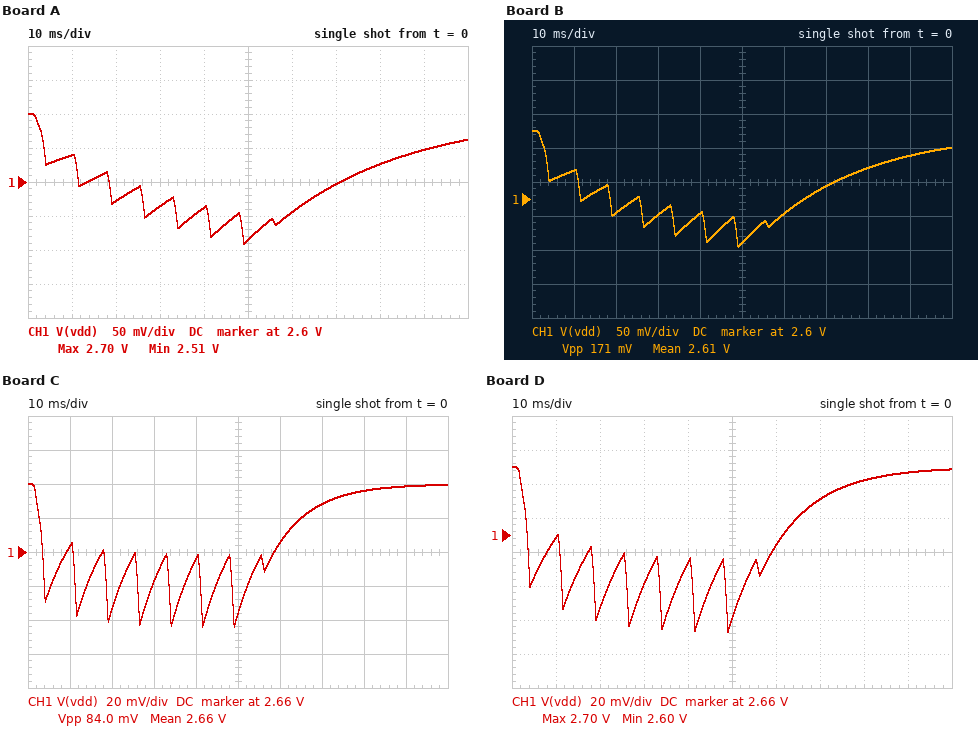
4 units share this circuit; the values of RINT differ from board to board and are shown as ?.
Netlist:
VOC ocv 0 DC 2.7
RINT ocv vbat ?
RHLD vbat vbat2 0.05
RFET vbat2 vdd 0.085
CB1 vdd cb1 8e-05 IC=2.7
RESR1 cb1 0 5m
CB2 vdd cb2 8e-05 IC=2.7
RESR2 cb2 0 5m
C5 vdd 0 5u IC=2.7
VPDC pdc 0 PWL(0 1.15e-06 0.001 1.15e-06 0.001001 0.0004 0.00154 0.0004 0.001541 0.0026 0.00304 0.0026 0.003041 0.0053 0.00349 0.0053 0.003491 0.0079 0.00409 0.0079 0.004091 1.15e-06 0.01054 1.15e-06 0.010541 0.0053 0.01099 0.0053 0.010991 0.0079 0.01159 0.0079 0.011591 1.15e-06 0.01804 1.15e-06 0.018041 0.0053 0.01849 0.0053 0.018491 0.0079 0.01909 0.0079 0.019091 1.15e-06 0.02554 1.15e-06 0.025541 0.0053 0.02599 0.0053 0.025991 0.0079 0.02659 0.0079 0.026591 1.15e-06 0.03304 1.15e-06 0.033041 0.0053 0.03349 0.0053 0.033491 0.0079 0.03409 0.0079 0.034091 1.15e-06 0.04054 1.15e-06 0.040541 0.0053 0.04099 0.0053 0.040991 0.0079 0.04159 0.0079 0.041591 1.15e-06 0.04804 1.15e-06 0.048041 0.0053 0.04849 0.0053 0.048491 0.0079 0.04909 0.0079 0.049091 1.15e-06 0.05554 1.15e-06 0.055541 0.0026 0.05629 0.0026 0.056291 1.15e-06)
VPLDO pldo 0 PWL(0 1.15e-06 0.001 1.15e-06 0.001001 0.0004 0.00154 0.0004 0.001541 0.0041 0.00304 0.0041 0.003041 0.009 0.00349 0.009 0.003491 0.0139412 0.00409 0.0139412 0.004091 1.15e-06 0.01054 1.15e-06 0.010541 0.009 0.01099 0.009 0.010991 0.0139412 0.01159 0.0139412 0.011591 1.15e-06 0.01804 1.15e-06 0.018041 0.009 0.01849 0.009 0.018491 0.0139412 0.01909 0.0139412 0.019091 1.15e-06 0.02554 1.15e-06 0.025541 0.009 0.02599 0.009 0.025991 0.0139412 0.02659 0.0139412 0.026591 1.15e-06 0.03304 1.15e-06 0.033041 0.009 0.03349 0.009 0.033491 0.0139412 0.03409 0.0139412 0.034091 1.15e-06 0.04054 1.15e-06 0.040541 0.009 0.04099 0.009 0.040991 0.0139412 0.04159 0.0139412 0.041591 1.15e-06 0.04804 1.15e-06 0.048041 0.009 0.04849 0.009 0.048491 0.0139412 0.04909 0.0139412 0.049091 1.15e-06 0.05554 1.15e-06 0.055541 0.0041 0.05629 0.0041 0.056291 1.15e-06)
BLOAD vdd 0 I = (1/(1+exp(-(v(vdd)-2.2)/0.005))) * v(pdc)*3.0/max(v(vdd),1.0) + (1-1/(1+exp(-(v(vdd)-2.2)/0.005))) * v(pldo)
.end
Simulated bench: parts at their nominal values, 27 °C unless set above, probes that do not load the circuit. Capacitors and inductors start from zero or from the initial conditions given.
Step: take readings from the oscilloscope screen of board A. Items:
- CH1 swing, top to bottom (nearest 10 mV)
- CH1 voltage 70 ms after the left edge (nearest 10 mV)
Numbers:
190 mV
2.60 V
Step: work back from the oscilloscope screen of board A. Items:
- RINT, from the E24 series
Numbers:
180 Ω
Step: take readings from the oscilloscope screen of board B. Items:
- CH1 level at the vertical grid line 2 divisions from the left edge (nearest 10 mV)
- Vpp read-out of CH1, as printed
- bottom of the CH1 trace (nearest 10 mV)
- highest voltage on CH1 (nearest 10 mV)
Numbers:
2.58 V
171 mV
2.53 V
2.70 V
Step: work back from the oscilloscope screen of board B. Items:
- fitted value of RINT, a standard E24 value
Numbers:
150 Ω
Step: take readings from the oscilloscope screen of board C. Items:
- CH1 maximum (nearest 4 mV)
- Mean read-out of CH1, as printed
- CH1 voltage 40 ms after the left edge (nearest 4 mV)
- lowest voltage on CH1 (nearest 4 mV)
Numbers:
2.700 V
2.66 V
2.656 V
2.616 V
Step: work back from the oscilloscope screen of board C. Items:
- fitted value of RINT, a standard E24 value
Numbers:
56 Ω
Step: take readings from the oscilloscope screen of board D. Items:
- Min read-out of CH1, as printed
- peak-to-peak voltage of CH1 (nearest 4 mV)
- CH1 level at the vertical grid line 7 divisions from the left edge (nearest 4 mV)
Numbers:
2.60 V
96 mV
2.680 V
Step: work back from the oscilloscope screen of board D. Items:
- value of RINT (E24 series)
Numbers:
68 Ω
